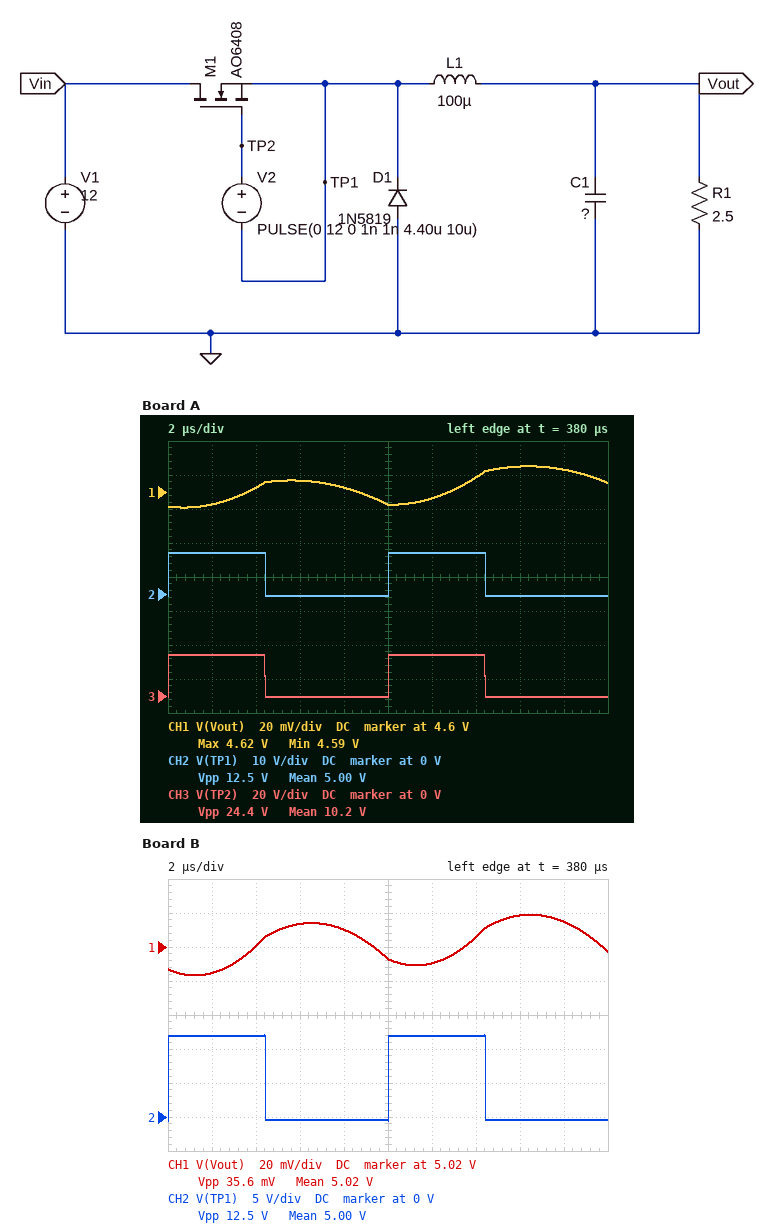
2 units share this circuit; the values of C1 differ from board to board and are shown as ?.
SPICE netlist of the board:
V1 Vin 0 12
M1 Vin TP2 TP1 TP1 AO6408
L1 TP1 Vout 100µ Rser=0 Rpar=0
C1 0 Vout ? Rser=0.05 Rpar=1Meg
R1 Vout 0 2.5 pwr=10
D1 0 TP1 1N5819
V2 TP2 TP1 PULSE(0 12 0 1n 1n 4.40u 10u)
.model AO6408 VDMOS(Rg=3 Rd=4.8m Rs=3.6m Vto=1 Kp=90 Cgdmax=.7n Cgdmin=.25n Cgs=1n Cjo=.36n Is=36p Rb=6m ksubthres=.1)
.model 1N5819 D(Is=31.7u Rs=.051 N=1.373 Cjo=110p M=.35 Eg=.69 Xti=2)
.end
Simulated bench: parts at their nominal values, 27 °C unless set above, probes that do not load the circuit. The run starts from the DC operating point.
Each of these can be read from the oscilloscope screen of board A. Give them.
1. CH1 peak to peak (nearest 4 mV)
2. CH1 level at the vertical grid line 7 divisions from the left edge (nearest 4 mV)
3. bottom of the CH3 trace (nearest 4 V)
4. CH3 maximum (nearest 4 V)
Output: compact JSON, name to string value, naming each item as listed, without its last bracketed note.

{"CH1 peak to peak": "24 mV", "CH1 level at the vertical grid line 7 divisions from the left edge": "4.608 V", "bottom of the CH3 trace": "0 V", "CH3 maximum": "24 V"}
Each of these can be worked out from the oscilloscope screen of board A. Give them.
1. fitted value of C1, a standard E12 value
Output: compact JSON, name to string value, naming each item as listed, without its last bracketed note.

{"fitted value of C1, a standard E12 value": "33 µF"}
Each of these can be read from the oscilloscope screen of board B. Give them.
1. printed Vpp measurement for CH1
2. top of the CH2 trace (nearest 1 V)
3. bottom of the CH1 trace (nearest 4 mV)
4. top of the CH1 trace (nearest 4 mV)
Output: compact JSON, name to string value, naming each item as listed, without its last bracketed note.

{"printed Vpp measurement for CH1": "35.6 mV", "top of the CH2 trace": "12 V", "bottom of the CH1 trace": "5.004 V", "top of the CH1 trace": "5.040 V"}
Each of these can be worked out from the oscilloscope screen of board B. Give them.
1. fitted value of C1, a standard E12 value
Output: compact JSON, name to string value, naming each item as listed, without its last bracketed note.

{"fitted value of C1, a standard E12 value": "15 µF"}
